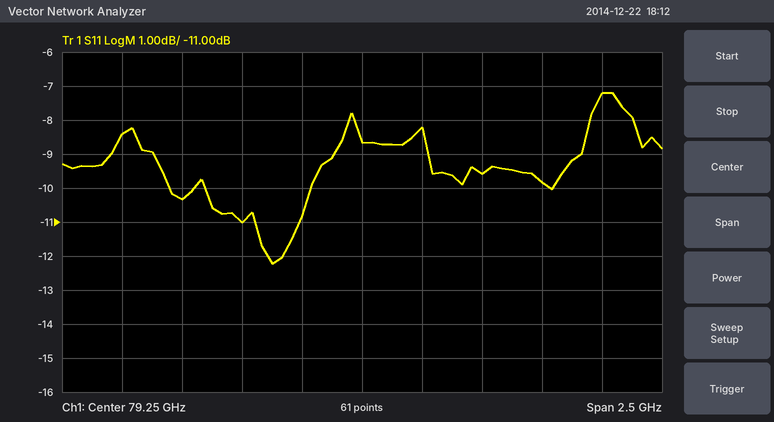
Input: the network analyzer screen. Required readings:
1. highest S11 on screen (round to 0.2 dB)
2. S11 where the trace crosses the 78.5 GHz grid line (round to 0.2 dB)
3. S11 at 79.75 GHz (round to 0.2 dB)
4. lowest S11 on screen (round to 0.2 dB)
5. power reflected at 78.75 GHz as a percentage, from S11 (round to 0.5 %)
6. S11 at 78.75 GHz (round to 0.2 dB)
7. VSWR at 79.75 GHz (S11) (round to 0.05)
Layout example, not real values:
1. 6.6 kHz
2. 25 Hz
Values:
1. -7.2 dB
2. -10.4 dB
3. -9.6 dB
4. -12.2 dB
5. 8.0 %
6. -11.0 dB
7. 2.00
